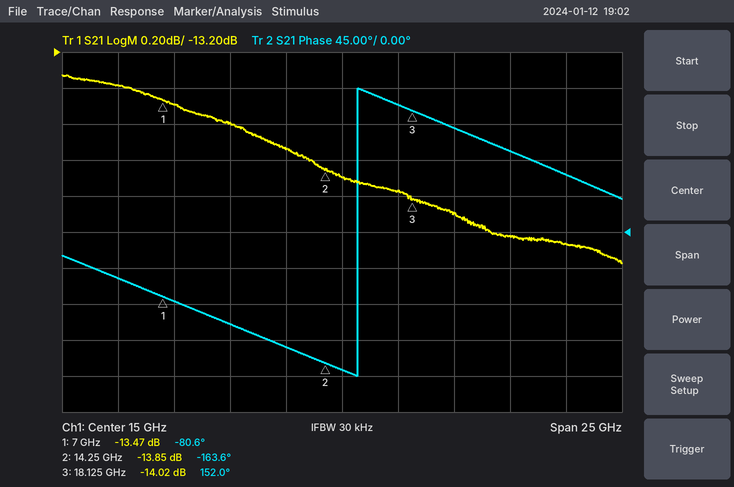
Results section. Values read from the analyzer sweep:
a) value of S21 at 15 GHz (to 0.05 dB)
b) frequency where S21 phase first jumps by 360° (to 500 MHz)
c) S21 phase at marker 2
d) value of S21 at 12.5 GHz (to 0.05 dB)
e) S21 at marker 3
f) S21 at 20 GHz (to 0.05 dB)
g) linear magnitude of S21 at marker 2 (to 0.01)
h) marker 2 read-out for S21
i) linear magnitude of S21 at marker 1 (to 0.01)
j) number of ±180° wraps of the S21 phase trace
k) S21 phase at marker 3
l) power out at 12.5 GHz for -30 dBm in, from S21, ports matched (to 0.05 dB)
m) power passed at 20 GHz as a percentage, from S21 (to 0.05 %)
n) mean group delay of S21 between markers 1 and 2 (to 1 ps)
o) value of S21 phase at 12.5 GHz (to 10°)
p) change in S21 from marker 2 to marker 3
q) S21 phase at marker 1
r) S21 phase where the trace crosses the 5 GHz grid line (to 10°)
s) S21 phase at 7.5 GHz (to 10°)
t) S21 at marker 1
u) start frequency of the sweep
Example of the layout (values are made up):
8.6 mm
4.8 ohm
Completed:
-13.90 dB
15.5 GHz
-163.6°
-13.75 dB
-14.02 dB
-14.10 dB
0.20
-13.85 dB
0.21
1
152.0°
-43.75 dBm
3.90 %
32 ps
-140°
-0.17 dB
-80.6°
-60°
-90°
-13.47 dB
2.5 GHz
